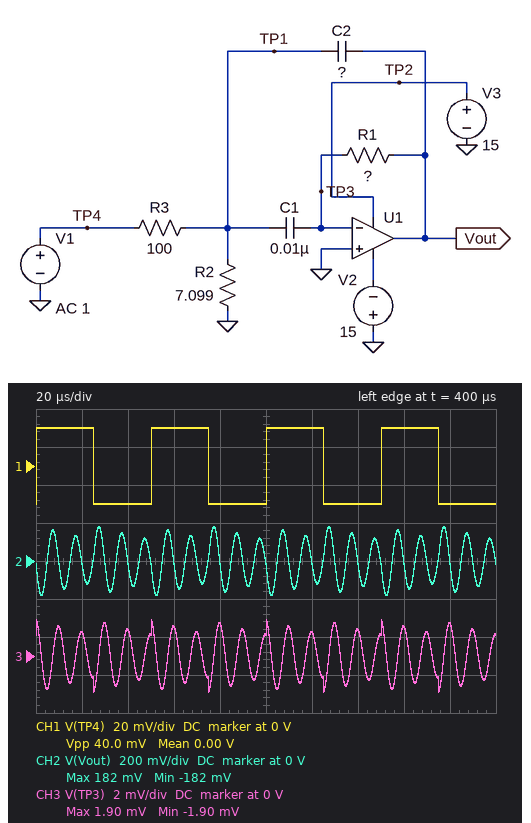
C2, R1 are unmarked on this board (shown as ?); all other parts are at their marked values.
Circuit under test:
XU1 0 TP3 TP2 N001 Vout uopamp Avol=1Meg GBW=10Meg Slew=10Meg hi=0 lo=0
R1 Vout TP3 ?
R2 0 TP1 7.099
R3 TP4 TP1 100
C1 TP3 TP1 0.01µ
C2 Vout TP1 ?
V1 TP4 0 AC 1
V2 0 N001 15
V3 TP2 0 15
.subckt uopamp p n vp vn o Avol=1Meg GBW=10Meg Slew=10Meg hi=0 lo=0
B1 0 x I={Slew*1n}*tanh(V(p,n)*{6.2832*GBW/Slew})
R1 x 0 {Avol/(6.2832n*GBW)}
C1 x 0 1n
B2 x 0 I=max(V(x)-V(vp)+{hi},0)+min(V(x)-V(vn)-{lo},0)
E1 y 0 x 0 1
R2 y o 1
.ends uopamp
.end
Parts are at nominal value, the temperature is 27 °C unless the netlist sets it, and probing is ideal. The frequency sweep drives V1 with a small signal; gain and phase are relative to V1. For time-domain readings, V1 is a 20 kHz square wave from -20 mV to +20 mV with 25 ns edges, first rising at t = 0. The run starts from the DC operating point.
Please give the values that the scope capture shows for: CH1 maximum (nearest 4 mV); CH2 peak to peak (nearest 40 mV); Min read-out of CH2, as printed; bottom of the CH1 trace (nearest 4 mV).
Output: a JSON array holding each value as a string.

["20 mV", "360 mV", "-182 mV", "-20 mV"]
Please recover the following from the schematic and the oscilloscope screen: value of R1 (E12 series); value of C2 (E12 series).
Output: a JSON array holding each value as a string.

["4.7 kΩ", "5.6 nF"]
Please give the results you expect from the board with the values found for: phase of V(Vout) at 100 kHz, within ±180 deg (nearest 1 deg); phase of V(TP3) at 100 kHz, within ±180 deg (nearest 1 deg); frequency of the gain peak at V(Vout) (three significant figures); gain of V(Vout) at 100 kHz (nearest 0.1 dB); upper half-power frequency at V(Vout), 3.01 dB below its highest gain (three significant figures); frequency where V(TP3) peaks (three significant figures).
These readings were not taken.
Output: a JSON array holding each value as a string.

["-167 deg", "103 deg", "101 kHz", "29.1 dB", "104 kHz", "101 kHz"]
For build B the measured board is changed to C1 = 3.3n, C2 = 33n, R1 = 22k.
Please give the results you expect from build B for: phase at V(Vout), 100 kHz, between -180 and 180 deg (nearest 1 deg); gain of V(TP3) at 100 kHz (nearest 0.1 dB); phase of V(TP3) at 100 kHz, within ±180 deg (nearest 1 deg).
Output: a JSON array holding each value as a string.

["91 deg", "-45.5 dB", "2 deg"]
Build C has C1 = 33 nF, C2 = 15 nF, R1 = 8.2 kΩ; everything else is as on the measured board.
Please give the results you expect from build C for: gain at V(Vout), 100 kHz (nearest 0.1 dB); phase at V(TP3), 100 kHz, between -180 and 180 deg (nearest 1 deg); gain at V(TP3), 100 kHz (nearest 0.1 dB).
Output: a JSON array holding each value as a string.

["0 dB", "1 deg", "-40.0 dB"]
